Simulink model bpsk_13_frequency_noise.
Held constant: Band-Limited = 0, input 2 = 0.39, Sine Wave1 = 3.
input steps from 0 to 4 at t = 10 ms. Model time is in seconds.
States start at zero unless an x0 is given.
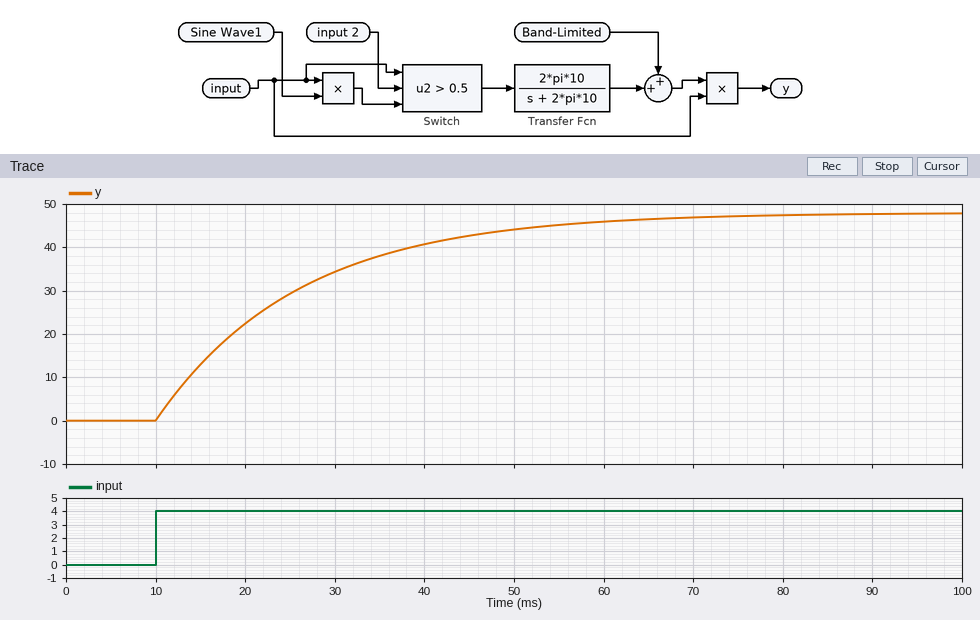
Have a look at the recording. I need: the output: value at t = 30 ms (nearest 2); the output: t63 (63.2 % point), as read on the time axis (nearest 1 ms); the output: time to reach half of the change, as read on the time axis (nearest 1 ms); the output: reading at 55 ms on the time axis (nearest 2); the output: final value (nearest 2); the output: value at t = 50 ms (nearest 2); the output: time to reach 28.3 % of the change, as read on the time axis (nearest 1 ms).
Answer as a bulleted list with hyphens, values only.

- 34
- 26 ms
- 21 ms
- 46
- 48
- 44
- 15 ms
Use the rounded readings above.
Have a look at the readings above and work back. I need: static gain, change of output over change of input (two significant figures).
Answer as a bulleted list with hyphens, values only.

- 12
